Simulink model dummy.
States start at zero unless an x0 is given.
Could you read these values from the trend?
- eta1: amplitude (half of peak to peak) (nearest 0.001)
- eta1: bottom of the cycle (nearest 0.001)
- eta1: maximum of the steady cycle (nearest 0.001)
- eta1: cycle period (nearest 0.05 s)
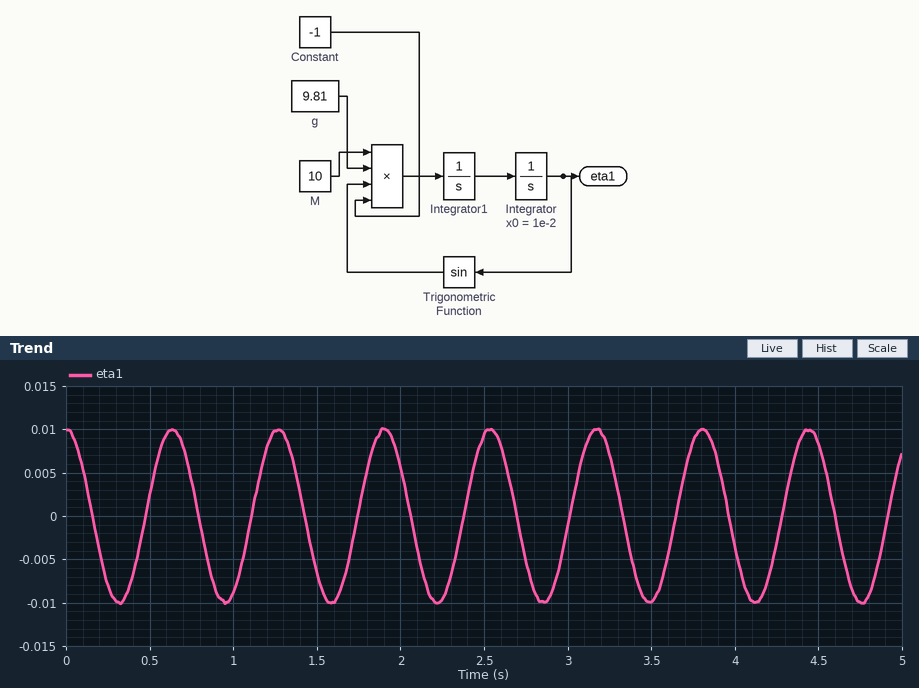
0.010
-0.010
0.010
0.65 s
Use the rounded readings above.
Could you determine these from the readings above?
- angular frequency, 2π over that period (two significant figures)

9.7 rad/s
